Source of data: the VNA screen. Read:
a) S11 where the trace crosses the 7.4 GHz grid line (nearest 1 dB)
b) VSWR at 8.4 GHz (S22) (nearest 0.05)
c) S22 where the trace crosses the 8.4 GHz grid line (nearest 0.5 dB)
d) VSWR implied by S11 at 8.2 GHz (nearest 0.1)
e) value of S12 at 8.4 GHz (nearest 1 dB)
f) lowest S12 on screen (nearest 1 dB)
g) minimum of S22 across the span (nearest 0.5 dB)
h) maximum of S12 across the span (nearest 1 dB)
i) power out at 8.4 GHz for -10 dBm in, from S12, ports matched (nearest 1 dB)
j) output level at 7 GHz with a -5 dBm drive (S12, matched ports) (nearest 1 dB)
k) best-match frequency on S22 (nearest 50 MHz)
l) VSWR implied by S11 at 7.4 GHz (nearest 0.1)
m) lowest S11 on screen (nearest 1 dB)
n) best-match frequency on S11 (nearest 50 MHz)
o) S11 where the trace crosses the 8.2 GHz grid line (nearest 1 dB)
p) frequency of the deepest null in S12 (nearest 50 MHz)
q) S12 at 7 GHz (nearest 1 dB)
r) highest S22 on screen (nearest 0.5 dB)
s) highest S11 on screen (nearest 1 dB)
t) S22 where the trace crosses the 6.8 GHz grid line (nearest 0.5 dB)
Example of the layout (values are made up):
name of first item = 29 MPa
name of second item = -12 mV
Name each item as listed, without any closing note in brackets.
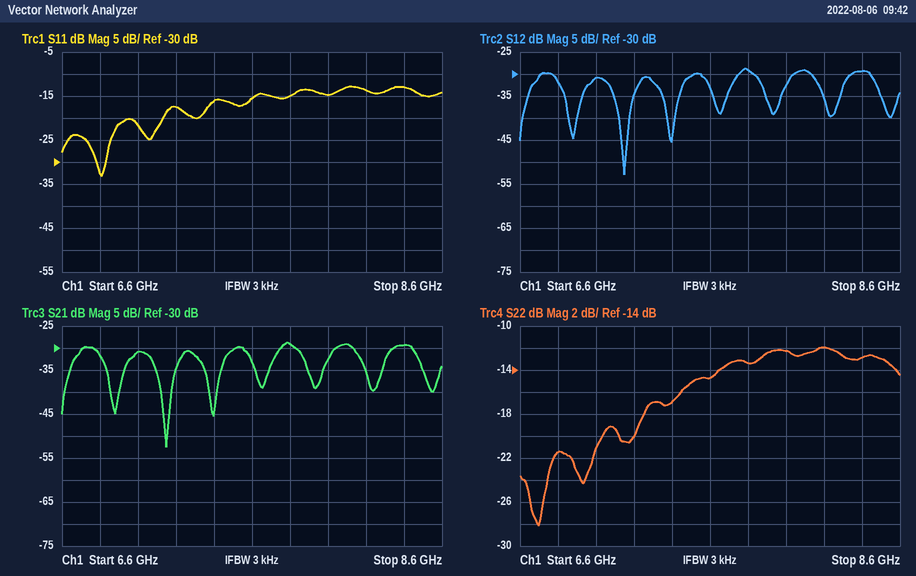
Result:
S11 where the trace crosses the 7.4 GHz grid line = -16 dB
VSWR at 8.4 GHz (S22) = 1.60
S22 where the trace crosses the 8.4 GHz grid line = -13.0 dB
VSWR implied by S11 at 8.2 GHz = 1.5
value of S12 at 8.4 GHz = -29 dB
lowest S12 on screen = -53 dB
minimum of S22 across the span = -28.0 dB
maximum of S12 across the span = -29 dB
power out at 8.4 GHz for -10 dBm in, from S12, ports matched = -39 dBm
output level at 7 GHz with a -5 dBm drive (S12, matched ports) = -36 dBm
best-match frequency on S22 = 6.70 GHz
VSWR implied by S11 at 7.4 GHz = 1.4
lowest S11 on screen = -33 dB
best-match frequency on S11 = 6.80 GHz
S11 where the trace crosses the 8.2 GHz grid line = -14 dB
frequency of the deepest null in S12 = 7.15 GHz
S12 at 7 GHz = -31 dB
highest S22 on screen = -12.0 dB
highest S11 on screen = -13 dB
S22 where the trace crosses the 6.8 GHz grid line = -21.5 dB
